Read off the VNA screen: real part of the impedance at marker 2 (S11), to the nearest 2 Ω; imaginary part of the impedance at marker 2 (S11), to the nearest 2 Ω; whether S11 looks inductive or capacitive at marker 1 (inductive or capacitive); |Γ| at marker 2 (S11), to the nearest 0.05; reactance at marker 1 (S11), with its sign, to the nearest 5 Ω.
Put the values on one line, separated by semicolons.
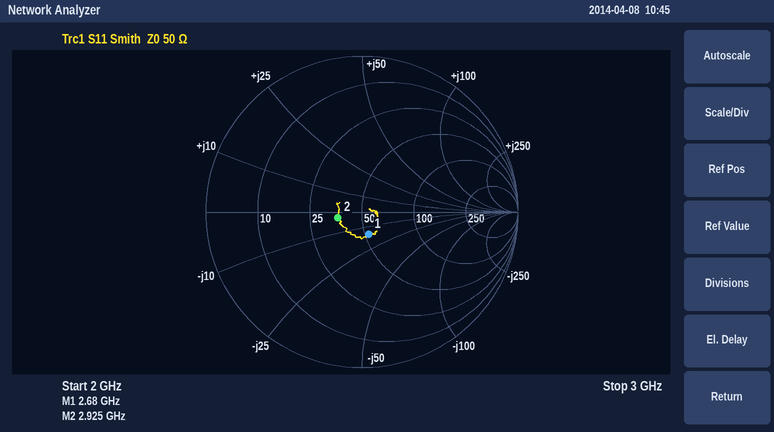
36 Ω; -2 Ω; capacitive; 0.15; -15 Ω
